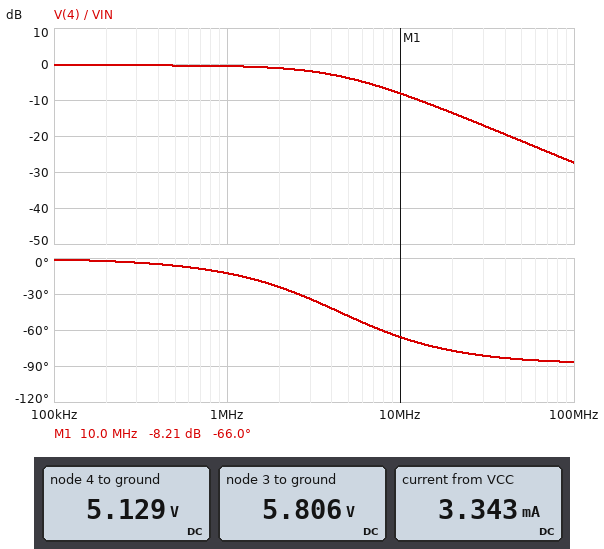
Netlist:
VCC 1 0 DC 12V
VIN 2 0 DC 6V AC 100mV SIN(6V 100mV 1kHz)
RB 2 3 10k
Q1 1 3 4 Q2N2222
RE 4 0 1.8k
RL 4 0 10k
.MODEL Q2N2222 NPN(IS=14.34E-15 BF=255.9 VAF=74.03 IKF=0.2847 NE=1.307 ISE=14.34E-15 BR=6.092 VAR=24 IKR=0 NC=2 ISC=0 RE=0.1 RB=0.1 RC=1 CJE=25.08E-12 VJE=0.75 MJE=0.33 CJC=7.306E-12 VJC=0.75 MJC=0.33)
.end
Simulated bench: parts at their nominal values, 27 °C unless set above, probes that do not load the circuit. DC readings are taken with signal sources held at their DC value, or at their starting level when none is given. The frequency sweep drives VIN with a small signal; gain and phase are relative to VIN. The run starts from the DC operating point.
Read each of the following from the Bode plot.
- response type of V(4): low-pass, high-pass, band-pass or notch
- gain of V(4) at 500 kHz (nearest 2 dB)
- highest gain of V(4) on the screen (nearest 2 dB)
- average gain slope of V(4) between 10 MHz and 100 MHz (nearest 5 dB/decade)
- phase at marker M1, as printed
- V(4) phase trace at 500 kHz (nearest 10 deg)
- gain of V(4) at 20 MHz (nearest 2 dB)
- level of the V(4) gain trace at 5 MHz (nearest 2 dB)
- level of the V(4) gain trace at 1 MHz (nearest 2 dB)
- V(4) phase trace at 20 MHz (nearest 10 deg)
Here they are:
low-pass
0 dB
0 dB
-20 dB/decade
-66.0 deg
-10 deg
-14 dB
-4 dB
0 dB
-80 deg
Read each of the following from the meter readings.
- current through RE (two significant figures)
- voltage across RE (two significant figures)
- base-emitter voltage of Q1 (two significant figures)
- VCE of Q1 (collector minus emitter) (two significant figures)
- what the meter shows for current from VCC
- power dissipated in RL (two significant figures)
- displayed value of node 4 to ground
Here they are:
2.8 mA
5.1 V
680 mV
6.9 V
3.343 mA
2.6 mW
5.129 V
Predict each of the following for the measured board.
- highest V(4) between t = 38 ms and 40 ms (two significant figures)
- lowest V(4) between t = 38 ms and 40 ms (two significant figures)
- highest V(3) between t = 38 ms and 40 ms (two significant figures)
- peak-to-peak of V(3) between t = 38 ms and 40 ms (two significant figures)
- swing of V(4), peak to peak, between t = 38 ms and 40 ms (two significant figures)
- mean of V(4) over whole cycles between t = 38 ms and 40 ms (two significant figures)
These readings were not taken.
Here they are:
5.2 V
5.0 V
5.9 V
190 mV
190 mV
5.1 V
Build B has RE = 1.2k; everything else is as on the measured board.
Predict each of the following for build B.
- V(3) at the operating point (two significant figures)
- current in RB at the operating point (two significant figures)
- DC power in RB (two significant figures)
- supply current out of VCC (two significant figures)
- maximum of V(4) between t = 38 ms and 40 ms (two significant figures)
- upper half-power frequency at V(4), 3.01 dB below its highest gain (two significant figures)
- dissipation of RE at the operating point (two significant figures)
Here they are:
5.7 V
27 µA
7.1 µW
4.7 mA
5.1 V
4.5 MHz
21 mW
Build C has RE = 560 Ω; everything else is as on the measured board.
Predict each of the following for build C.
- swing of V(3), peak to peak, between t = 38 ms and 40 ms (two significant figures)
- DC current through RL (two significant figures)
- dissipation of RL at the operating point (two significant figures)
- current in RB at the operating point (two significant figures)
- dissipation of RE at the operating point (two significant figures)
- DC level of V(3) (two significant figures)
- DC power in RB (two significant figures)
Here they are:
180 mV
480 µA
2.3 mW
49 µA
41 mW
5.5 V
24 µW
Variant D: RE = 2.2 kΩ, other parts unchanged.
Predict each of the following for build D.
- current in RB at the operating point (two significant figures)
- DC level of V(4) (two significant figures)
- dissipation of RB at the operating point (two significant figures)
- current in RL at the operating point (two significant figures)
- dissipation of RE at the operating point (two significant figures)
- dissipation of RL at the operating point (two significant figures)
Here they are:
17 µA
5.2 V
2.8 µW
520 µA
12 mW
2.7 mW
